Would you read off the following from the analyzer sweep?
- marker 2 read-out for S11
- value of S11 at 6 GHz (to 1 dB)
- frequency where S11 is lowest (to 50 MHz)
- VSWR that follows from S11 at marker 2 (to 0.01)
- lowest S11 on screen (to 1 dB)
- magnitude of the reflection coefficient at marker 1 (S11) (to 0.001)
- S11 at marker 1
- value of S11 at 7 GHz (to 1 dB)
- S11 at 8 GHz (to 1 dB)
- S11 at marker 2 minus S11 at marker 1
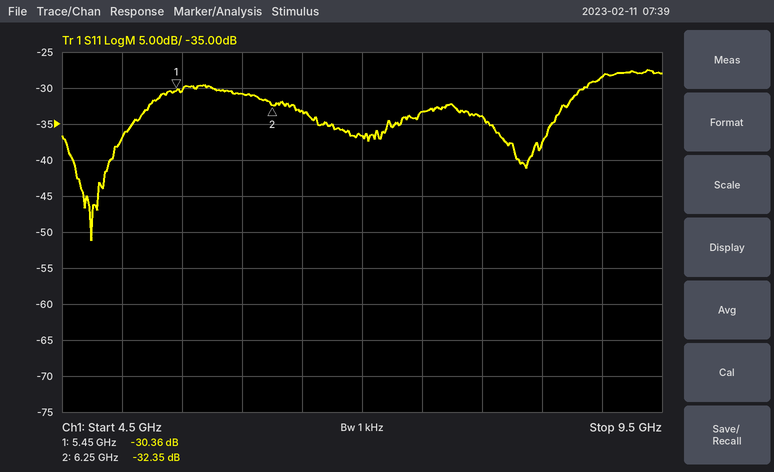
-32.35 dB
-31 dB
4.75 GHz
1.05
-51 dB
0.030
-30.36 dB
-37 dB
-34 dB
-1.99 dB
